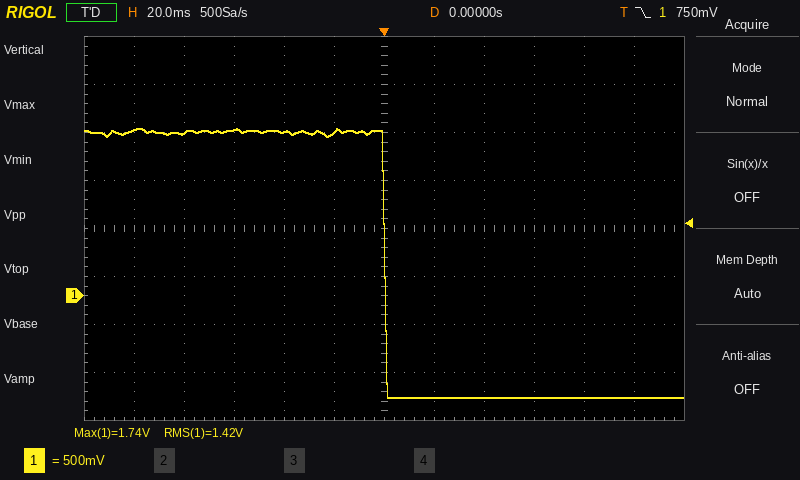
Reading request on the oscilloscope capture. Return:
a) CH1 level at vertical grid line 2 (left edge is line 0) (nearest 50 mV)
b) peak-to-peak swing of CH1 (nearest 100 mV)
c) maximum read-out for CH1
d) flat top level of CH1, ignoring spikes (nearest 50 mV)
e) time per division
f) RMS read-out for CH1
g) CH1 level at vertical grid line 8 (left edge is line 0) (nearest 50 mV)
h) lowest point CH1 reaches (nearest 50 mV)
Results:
1.70 V
2.80 V
1.74 V
1.70 V
20 ms
1.42 V
-1.05 V
-1.05 V
